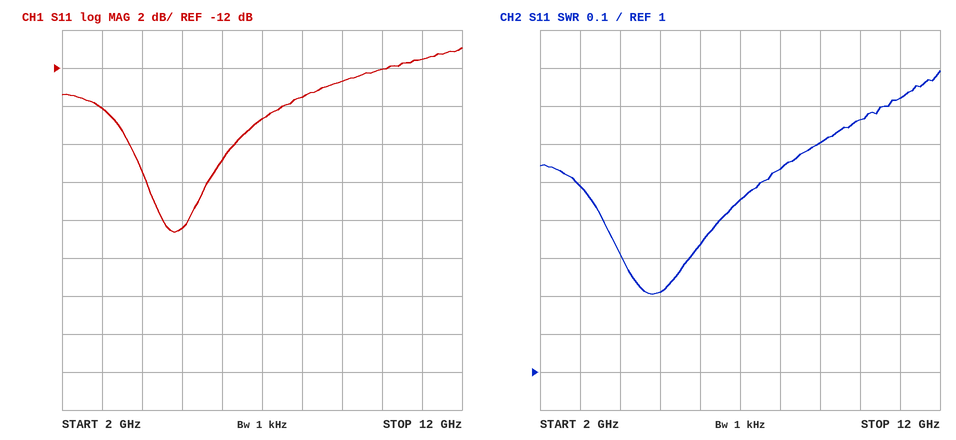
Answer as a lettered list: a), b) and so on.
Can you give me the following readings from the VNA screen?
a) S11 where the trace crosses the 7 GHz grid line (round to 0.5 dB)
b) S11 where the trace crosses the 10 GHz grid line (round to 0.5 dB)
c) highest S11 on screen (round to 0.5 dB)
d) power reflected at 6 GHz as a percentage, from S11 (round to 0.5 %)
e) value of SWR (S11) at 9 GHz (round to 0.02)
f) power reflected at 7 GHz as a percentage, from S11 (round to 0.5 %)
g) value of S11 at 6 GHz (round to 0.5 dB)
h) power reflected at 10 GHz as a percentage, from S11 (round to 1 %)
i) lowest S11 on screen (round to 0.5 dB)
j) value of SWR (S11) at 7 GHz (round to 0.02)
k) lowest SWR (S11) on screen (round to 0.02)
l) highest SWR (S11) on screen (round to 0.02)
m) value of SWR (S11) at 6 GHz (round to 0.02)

a) -14.5 dB
b) -12.0 dB
c) -11.0 dB
d) 2.0 %
e) 1.60
f) 3.5 %
g) -17.0 dB
h) 6 %
i) -20.5 dB
j) 1.46
k) 1.20
l) 1.80
m) 1.34
